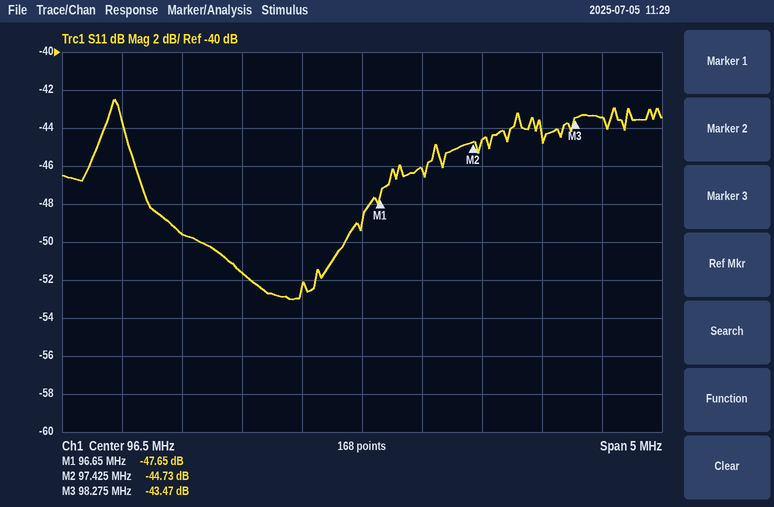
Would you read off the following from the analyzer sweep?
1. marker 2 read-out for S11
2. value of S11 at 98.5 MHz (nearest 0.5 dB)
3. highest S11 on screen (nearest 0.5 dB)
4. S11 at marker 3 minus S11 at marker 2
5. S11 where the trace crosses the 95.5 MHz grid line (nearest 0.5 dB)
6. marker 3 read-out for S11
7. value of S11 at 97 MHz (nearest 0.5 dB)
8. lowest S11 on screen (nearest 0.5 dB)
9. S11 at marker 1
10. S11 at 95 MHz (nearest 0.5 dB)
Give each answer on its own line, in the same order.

-44.73 dB
-43.5 dB
-42.5 dB
1.26 dB
-51.5 dB
-43.47 dB
-46.0 dB
-53.0 dB
-47.65 dB
-49.5 dB
